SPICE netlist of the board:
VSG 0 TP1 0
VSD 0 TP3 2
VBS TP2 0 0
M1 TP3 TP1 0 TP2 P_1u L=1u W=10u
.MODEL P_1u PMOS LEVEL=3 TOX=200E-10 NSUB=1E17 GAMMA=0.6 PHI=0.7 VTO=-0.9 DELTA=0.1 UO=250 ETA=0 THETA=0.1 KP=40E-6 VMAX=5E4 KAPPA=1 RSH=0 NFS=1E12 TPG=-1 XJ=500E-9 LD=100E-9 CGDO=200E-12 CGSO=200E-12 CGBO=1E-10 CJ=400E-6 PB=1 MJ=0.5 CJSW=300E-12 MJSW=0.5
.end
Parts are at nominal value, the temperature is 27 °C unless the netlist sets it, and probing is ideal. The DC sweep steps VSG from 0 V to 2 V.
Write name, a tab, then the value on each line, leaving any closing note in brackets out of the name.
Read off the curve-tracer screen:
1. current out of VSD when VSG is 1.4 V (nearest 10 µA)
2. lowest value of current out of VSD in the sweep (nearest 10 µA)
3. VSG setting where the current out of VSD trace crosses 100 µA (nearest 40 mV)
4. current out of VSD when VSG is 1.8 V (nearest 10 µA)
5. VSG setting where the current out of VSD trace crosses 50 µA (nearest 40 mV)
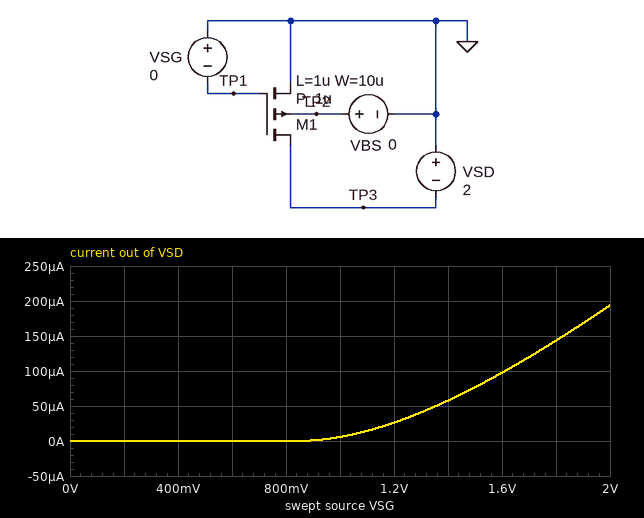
current out of VSD when VSG is 1.4 V	60 µA
lowest value of current out of VSD in the sweep	0 A
VSG setting where the current out of VSD trace crosses 100 µA	1.60 V
current out of VSD when VSG is 1.8 V	140 µA
VSG setting where the current out of VSD trace crosses 50 µA	1.36 V
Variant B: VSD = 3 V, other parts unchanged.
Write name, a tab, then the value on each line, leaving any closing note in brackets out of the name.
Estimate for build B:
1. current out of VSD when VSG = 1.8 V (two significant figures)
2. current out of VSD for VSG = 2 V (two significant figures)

current out of VSD when VSG = 1.8 V	150 µA
current out of VSD for VSG = 2 V	210 µA
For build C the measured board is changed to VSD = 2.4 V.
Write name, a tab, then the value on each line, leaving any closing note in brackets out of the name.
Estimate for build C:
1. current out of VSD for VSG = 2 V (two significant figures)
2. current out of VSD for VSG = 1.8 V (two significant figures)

current out of VSD for VSG = 2 V	200 µA
current out of VSD for VSG = 1.8 V	150 µA
